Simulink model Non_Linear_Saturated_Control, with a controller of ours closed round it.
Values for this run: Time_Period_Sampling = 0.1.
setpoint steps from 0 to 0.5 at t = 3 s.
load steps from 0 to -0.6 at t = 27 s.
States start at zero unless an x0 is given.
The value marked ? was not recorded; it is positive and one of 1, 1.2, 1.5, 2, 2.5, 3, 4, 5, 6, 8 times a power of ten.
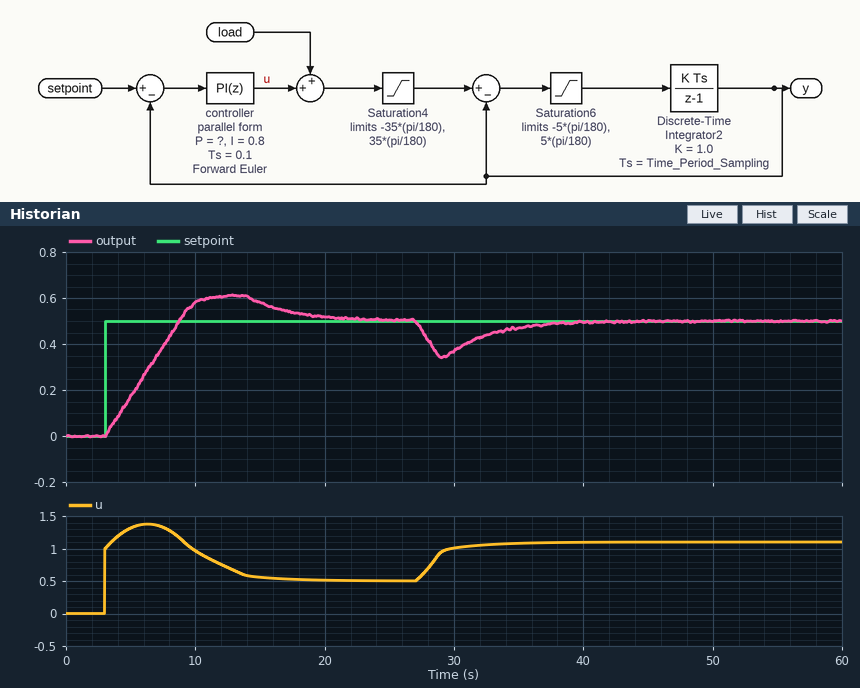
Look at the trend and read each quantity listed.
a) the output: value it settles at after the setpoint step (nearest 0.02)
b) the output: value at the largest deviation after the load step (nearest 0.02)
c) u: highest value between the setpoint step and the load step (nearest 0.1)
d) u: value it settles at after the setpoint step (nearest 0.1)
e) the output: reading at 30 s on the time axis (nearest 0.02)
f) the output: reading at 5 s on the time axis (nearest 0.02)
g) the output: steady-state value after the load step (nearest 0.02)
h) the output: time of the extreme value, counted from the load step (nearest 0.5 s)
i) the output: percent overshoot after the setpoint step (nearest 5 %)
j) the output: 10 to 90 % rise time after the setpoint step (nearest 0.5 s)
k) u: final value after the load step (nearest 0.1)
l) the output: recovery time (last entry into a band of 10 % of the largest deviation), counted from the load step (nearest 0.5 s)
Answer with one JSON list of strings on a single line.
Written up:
["0.50", "0.34", "1.4", "0.5", "0.38", "0.18", "0.50", "2.0 s", "20 %", "4.5 s", "1.1", "10.0 s"]
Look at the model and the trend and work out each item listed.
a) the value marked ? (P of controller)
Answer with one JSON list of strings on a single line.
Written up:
["2"]
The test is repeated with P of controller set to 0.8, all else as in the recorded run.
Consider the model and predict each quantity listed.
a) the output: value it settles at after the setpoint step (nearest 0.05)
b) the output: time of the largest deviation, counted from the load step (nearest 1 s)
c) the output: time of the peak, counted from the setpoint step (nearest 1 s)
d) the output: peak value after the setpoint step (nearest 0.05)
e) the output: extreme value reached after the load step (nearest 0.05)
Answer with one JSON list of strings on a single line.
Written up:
["0.50", "3 s", "12 s", "0.60", "0.30"]
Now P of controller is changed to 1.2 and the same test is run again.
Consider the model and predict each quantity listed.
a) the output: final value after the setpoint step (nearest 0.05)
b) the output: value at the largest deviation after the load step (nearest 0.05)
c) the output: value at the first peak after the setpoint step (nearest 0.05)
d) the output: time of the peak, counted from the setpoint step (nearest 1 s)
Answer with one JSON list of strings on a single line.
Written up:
["0.50", "0.30", "0.60", "12 s"]
